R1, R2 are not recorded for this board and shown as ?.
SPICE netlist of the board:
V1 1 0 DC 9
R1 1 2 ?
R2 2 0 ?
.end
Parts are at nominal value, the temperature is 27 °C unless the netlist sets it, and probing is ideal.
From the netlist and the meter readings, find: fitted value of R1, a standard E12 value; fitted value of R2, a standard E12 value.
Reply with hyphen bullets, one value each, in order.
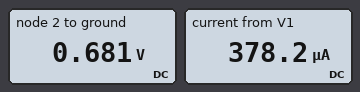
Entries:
- 22 kΩ
- 1.8 kΩ
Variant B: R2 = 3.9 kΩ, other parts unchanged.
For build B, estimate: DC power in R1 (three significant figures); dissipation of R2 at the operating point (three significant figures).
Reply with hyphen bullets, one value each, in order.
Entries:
- 2.66 mW
- 471 µW
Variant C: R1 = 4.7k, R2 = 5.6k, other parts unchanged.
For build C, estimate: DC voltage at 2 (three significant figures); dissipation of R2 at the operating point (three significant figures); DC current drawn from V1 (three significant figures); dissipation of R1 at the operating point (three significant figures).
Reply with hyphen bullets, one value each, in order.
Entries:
- 4.89 V
- 4.28 mW
- 874 µA
- 3.59 mW
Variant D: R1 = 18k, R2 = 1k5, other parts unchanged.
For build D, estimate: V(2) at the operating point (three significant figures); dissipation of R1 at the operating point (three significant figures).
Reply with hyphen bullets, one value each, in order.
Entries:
- 692 mV
- 3.83 mW
